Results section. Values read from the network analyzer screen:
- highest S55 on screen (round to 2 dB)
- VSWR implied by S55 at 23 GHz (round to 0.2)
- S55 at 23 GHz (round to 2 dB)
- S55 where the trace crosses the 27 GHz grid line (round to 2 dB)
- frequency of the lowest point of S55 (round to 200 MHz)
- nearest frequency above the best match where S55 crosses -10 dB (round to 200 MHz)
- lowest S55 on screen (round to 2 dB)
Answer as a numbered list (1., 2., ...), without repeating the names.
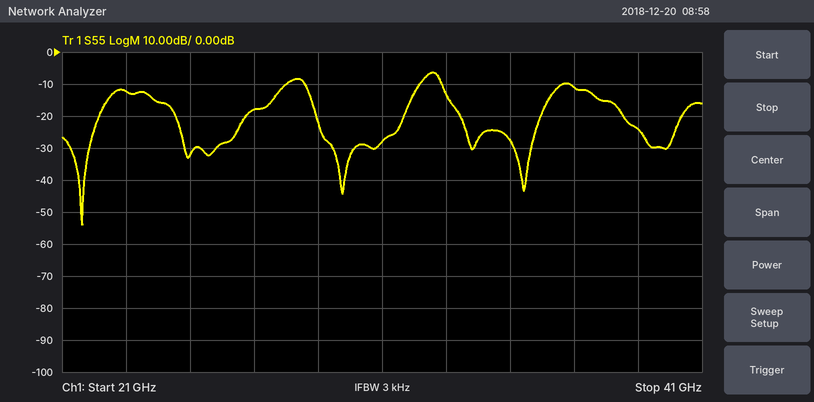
1. -6 dB
2. 1.6
3. -12 dB
4. -18 dB
5. 21.6 GHz
6. 28.0 GHz
7. -54 dB
